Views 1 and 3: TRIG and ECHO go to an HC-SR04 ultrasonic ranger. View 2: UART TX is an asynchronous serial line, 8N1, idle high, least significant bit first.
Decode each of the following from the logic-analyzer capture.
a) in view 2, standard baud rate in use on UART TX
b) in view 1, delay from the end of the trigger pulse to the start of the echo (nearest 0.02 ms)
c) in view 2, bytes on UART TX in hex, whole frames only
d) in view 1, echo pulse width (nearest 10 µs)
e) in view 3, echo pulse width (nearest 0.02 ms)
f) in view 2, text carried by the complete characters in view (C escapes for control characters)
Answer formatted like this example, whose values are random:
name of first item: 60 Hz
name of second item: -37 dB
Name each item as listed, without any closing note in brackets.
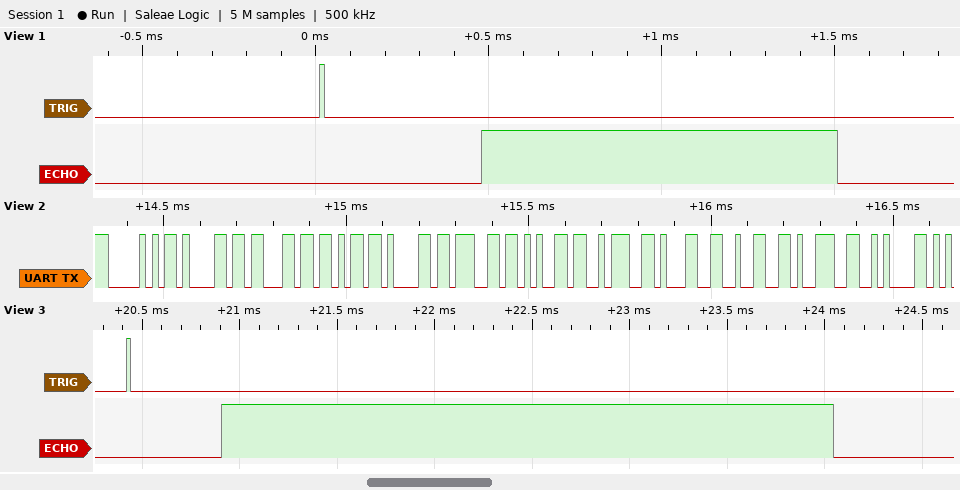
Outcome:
in view 2, standard baud rate in use on UART TX: 57600 baud
in view 1, delay from the end of the trigger pulse to the start of the echo: 0.46 ms
in view 2, bytes on UART TX in hex, whole frames only: 50 61 63 6B 61 67 65 3A 31 32 39 0A
in view 1, echo pulse width: 1030 µs
in view 3, echo pulse width: 3.14 ms
in view 2, text carried by the complete characters in view: "Package:129\n"
